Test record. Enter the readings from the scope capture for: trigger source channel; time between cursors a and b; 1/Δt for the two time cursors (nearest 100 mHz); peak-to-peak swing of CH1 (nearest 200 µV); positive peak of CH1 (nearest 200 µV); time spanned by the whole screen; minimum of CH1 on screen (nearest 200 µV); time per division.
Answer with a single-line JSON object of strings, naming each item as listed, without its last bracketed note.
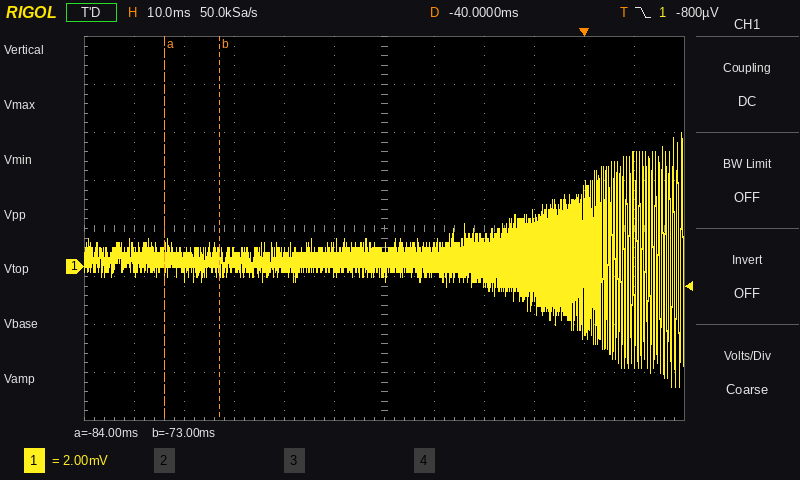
{"trigger source channel": "CH1", "time between cursors a and b": "11 ms", "1/Δt for the two time cursors": "90.9 Hz", "peak-to-peak swing of CH1": "10.6 mV", "positive peak of CH1": "5.6 mV", "time spanned by the whole screen": "120 ms", "minimum of CH1 on screen": "-5.0 mV", "time per division": "10 ms"}
